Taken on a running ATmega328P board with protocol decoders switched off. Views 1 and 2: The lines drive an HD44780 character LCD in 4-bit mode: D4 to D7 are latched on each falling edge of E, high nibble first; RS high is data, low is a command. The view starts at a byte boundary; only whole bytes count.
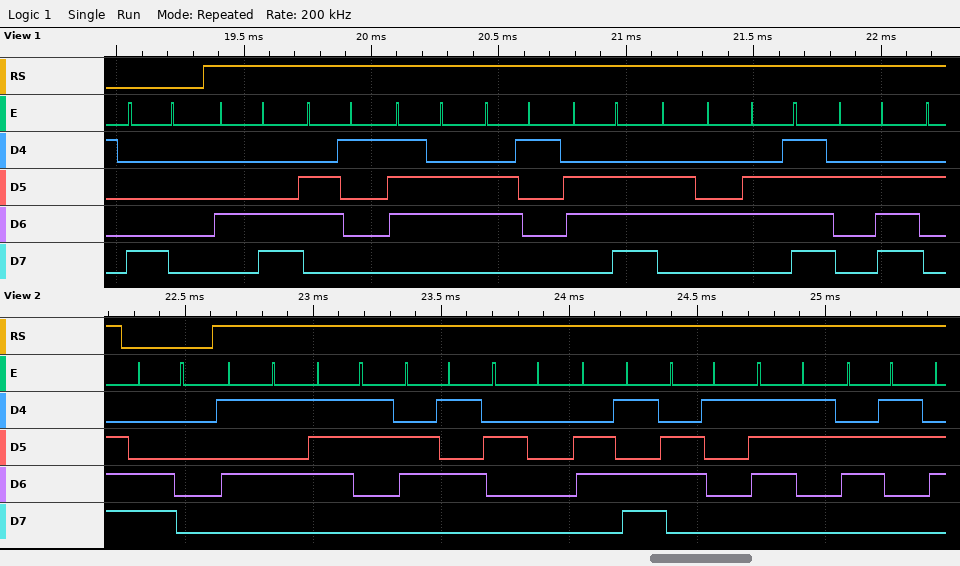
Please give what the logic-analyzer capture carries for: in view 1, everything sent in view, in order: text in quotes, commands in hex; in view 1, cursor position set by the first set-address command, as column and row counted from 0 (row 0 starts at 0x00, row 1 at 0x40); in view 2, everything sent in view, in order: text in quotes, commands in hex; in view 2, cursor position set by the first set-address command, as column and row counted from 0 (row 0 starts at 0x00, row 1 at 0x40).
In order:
0x80 "Lavando."
column 0, row 0
0xC0 "Use masc"
column 0, row 1
